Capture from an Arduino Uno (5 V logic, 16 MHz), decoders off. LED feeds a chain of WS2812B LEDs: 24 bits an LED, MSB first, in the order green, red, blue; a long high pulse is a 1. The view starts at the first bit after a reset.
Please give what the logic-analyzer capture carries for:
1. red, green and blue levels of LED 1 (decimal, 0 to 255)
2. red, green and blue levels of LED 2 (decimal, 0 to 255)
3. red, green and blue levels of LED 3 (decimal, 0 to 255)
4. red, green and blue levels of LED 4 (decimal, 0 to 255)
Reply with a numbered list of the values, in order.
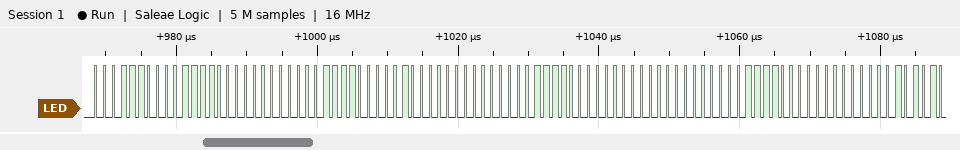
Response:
1. 60, 28, 0
2. 16, 60, 0
3. 0, 60, 0
4. 0, 60, 21
